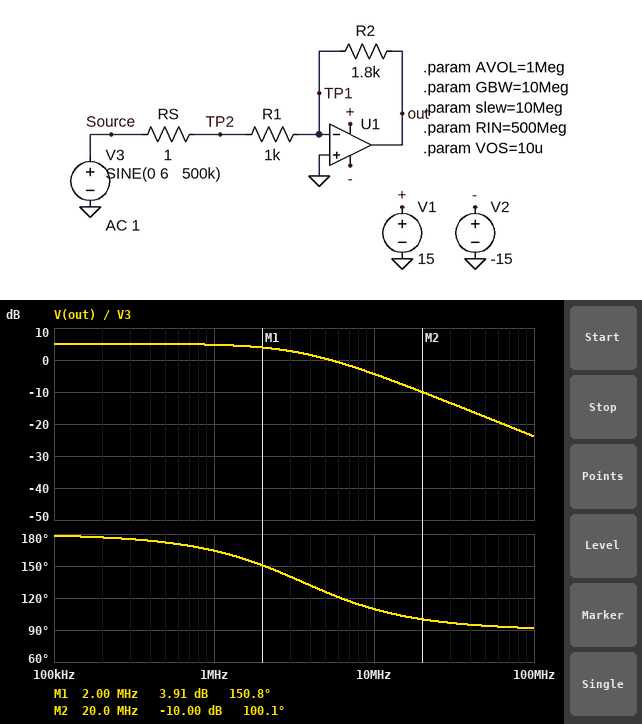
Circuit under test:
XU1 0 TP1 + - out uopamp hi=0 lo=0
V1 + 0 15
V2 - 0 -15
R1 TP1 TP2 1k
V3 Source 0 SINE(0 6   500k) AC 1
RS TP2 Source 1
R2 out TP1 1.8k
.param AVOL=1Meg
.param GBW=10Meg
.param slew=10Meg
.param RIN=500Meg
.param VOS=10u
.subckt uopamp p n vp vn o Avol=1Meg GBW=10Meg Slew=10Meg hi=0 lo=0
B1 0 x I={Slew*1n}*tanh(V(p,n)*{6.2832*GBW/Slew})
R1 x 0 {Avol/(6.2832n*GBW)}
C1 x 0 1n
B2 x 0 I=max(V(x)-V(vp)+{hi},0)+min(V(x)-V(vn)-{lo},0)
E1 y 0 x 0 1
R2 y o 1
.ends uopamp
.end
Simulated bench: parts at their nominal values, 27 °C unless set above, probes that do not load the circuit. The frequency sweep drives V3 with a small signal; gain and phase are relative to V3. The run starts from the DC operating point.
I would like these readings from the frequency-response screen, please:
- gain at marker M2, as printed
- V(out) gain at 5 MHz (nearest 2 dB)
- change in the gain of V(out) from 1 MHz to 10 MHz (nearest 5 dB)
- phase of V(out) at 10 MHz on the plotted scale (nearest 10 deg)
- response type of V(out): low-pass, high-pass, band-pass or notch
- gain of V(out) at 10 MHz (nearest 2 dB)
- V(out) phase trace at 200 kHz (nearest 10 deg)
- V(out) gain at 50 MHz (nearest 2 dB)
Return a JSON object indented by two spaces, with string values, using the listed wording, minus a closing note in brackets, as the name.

{
  "gain at marker M2, as printed": "-10.00 dB",
  "V(out) gain at 5 MHz": "0 dB",
  "change in the gain of V(out) from 1 MHz to 10 MHz": "-10 dB",
  "phase of V(out) at 10 MHz on the plotted scale": "110 deg",
  "response type of V(out): low-pass, high-pass, band-pass or notch": "low-pass",
  "gain of V(out) at 10 MHz": "-4 dB",
  "V(out) phase trace at 200 kHz": "180 deg",
  "V(out) gain at 50 MHz": "-18 dB"
}
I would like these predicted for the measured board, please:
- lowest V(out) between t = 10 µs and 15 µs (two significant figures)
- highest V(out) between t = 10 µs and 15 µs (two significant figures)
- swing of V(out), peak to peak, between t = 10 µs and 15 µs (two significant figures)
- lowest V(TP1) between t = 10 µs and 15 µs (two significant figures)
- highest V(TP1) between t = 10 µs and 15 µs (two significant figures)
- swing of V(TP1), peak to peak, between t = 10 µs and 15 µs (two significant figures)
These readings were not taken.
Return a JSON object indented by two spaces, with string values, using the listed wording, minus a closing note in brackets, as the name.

{
  "lowest V(out) between t = 10 µs and 15 µs": "-4.9 V",
  "highest V(out) between t = 10 µs and 15 µs": "4.9 V",
  "swing of V(out), peak to peak, between t = 10 µs and 15 µs": "9.8 V",
  "lowest V(TP1) between t = 10 µs and 15 µs": "-3.5 V",
  "highest V(TP1) between t = 10 µs and 15 µs": "3.5 V",
  "swing of V(TP1), peak to peak, between t = 10 µs and 15 µs": "7.0 V"
}
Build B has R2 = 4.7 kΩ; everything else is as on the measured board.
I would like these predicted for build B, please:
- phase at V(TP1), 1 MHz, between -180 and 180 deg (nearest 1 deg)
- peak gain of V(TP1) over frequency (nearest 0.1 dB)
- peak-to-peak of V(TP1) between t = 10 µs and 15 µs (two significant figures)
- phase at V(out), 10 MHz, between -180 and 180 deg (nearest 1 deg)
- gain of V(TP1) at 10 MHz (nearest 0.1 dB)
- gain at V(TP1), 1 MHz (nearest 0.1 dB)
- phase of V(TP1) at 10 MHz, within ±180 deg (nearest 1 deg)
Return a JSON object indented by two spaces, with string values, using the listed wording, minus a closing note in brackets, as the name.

{
  "phase at V(TP1), 1 MHz, between -180 and 180 deg": "60 deg",
  "peak gain of V(TP1) over frequency": "-1.7 dB",
  "peak-to-peak of V(TP1) between t = 10 µs and 15 µs": "9.8 V",
  "phase at V(out), 10 MHz, between -180 and 180 deg": "100 deg",
  "gain of V(TP1) at 10 MHz": "-1.8 dB",
  "gain at V(TP1), 1 MHz": "-7.8 dB",
  "phase of V(TP1) at 10 MHz, within ±180 deg": "10 deg"
}
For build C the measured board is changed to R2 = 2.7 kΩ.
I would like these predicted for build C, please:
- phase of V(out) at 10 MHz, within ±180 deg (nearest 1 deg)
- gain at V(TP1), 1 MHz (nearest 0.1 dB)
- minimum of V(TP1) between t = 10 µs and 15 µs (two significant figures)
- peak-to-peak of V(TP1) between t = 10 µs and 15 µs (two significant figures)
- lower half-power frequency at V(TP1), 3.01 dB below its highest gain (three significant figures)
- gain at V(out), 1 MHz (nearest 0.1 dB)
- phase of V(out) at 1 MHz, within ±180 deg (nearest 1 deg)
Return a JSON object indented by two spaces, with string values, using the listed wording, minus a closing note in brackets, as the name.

{
  "phase of V(out) at 10 MHz, within ±180 deg": "105 deg",
  "gain at V(TP1), 1 MHz": "-11.9 dB",
  "minimum of V(TP1) between t = 10 µs and 15 µs": "-4.2 V",
  "peak-to-peak of V(TP1) between t = 10 µs and 15 µs": "8.4 V",
  "lower half-power frequency at V(TP1), 3.01 dB below its highest gain": "2.70 MHz",
  "gain at V(out), 1 MHz": "8.1 dB",
  "phase of V(out) at 1 MHz, within ±180 deg": "160 deg"
}
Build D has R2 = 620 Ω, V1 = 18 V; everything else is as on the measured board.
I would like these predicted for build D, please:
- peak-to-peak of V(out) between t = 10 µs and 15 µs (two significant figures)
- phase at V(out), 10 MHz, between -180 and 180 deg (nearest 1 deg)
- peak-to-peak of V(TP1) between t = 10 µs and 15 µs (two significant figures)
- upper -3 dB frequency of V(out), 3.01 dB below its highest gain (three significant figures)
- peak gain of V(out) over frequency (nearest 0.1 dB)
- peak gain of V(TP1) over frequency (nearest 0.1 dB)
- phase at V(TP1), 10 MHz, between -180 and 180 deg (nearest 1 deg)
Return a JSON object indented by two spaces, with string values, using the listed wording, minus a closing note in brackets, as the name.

{
  "peak-to-peak of V(out) between t = 10 µs and 15 µs": "7.4 V",
  "phase at V(out), 10 MHz, between -180 and 180 deg": "122 deg",
  "peak-to-peak of V(TP1) between t = 10 µs and 15 µs": "1.0 V",
  "upper -3 dB frequency of V(out), 3.01 dB below its highest gain": "6.17 MHz",
  "peak gain of V(out) over frequency": "-4.2 dB",
  "peak gain of V(TP1) over frequency": "-8.3 dB",
  "phase at V(TP1), 10 MHz, between -180 and 180 deg": "32 deg"
}
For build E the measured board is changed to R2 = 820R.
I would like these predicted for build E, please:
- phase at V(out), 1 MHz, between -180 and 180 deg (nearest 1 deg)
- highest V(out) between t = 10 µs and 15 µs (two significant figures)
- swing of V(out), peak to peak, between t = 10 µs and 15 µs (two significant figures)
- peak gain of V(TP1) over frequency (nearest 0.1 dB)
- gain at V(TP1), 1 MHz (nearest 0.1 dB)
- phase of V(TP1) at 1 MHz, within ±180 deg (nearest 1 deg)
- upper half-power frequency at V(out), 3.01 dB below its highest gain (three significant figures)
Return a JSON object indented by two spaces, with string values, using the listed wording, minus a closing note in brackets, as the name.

{
  "phase at V(out), 1 MHz, between -180 and 180 deg": "170 deg",
  "highest V(out) between t = 10 µs and 15 µs": "4.6 V",
  "swing of V(out), peak to peak, between t = 10 µs and 15 µs": "9.1 V",
  "peak gain of V(TP1) over frequency": "-6.9 dB",
  "gain at V(TP1), 1 MHz": "-21.9 dB",
  "phase of V(TP1) at 1 MHz, within ±180 deg": "80 deg",
  "upper half-power frequency at V(out), 3.01 dB below its highest gain": "5.49 MHz"
}
